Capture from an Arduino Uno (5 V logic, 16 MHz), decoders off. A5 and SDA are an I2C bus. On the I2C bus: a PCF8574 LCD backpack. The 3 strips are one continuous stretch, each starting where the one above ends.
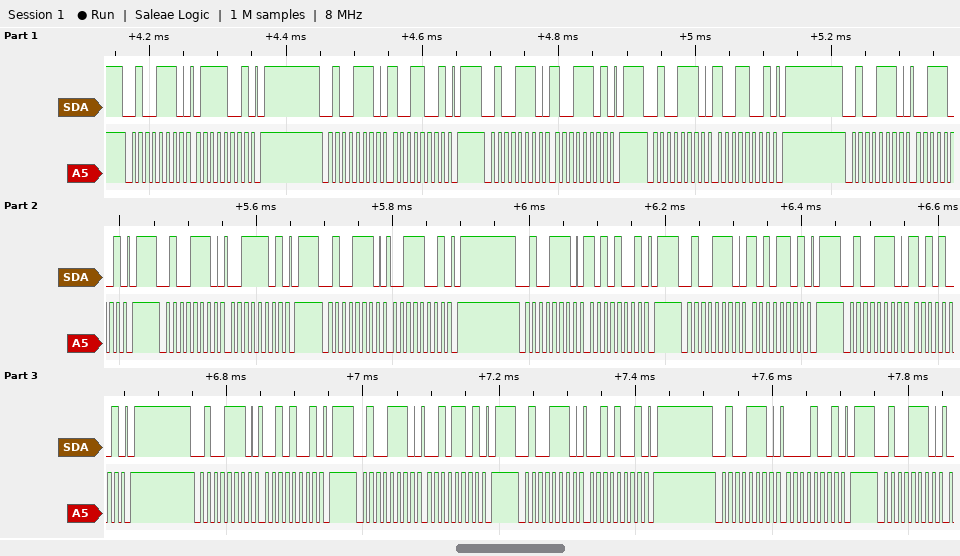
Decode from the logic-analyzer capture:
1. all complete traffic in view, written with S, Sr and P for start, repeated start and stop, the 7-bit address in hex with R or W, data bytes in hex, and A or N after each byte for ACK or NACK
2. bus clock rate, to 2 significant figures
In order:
S 27W A 79 A P S 27W A 99 A P S 27W A 9D A P S 27W A 99 A P S 27W A 39 A P S 27W A 3D A P S 27W A 39 A P S 27W A A9 A P S 27W A AD A P S 27W A A9 A P S 27W A 29 A P S 27W A 2D A P S 27W A 29 A P S 27W A 09 A P S 27W A
100 kHz
